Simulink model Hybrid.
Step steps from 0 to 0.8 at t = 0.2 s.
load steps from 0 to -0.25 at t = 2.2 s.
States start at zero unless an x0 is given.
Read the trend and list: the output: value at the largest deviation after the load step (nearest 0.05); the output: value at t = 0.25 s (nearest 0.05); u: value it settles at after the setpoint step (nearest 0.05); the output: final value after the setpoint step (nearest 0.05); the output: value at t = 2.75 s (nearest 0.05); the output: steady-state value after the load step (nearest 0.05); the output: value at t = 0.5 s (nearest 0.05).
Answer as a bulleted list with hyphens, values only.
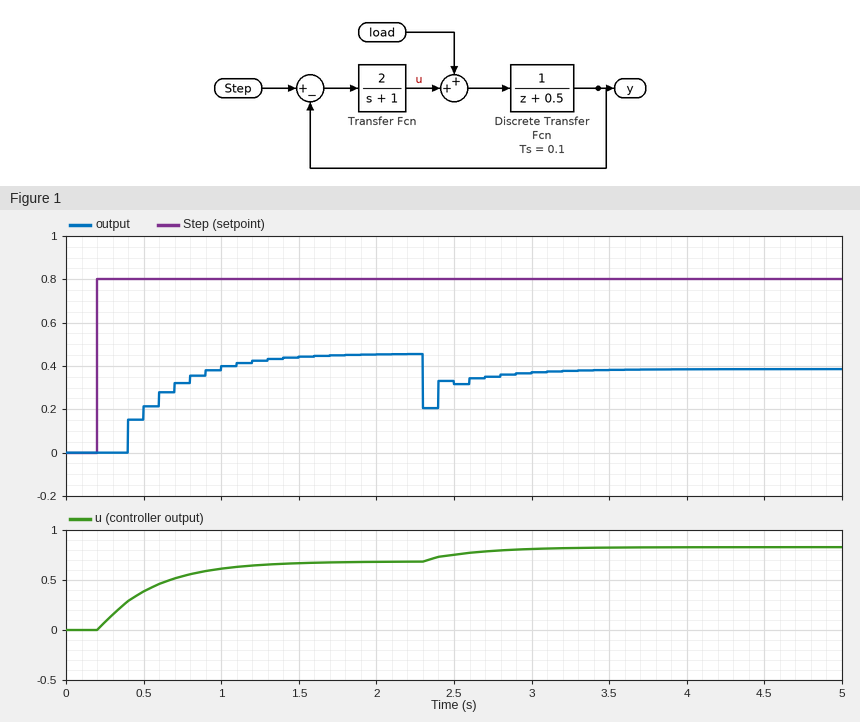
- 0.20
- 0.00
- 0.70
- 0.45
- 0.35
- 0.40
- 0.20
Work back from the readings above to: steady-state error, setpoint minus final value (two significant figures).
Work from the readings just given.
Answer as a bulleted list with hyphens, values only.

- 0.35
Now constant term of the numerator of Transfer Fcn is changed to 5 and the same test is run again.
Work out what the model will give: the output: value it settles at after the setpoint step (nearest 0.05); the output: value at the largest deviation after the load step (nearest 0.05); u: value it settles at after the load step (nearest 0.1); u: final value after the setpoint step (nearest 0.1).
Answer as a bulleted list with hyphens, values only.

- 0.60
- 0.35
- 1.1
- 0.9
